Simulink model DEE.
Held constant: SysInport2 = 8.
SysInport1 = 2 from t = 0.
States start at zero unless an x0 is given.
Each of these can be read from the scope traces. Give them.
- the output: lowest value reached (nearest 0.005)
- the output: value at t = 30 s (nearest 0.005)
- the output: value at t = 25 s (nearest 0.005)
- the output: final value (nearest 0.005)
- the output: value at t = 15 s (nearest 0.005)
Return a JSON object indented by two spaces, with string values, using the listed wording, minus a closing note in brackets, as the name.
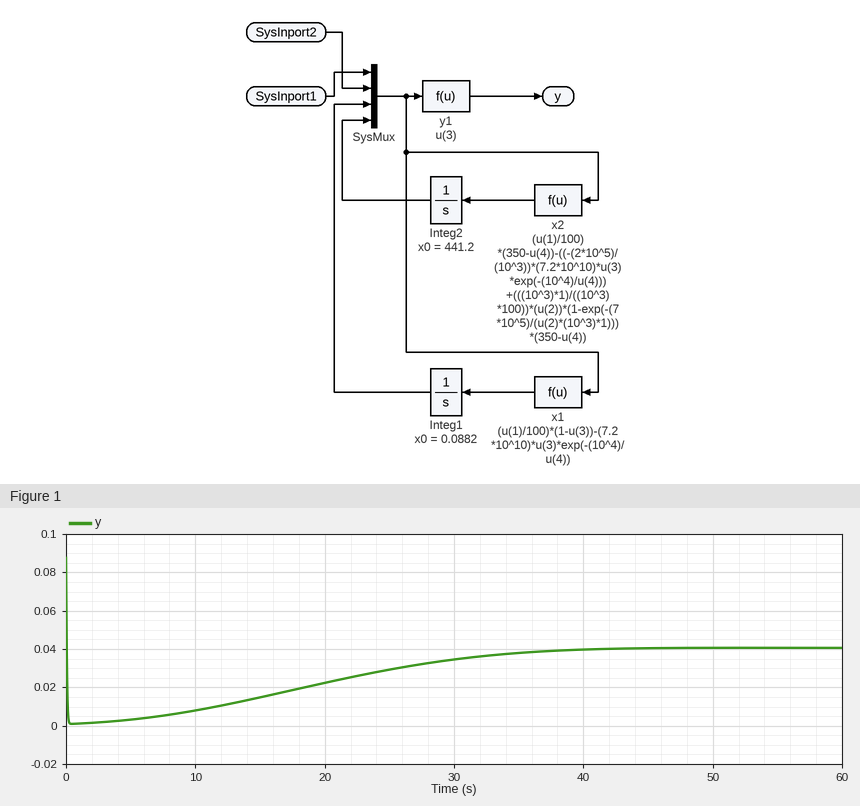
{
  "the output: lowest value reached": "0.000",
  "the output: value at t = 30 s": "0.035",
  "the output: value at t = 25 s": "0.030",
  "the output: final value": "0.040",
  "the output: value at t = 15 s": "0.015"
}
